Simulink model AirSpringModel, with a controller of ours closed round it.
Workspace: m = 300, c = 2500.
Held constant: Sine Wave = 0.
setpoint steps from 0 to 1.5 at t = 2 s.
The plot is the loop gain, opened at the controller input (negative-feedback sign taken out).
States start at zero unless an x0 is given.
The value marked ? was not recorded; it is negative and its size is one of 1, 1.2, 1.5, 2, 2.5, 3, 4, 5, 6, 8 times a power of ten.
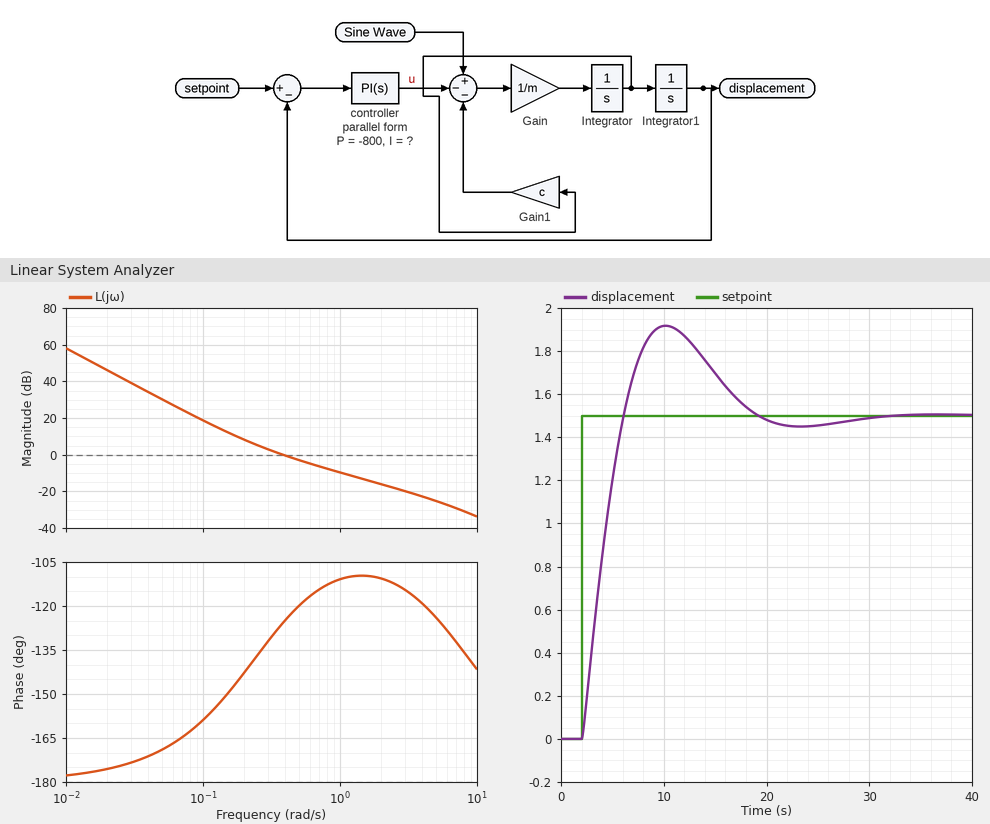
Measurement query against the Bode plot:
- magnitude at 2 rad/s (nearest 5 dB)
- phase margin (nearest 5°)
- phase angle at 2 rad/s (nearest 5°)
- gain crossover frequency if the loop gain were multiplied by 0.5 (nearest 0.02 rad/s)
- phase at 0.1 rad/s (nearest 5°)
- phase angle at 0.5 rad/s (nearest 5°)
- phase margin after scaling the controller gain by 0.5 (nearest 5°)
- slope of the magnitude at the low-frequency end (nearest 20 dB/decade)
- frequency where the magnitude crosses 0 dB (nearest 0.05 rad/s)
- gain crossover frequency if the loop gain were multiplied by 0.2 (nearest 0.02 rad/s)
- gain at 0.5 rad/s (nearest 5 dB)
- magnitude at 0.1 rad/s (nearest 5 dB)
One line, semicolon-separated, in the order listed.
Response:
-15 dB; 55°; -110°; 0.24 rad/s; -160°; -120°; 40°; -40 dB/decade; 0.40 rad/s; 0.14 rad/s; -5 dB; 20 dB
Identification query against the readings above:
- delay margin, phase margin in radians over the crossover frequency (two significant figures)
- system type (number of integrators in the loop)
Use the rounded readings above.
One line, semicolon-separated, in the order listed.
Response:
2.4 s; 2
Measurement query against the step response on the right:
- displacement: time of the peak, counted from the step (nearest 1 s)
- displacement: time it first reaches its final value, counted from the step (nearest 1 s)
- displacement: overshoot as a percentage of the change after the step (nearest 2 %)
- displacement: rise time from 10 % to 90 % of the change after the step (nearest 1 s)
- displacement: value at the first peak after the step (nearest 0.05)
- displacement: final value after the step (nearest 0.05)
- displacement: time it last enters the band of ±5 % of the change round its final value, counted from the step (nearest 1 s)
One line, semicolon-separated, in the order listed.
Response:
8 s; 4 s; 28 %; 3 s; 1.90; 1.50; 15 s
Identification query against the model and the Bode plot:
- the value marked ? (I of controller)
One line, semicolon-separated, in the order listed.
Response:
-200
